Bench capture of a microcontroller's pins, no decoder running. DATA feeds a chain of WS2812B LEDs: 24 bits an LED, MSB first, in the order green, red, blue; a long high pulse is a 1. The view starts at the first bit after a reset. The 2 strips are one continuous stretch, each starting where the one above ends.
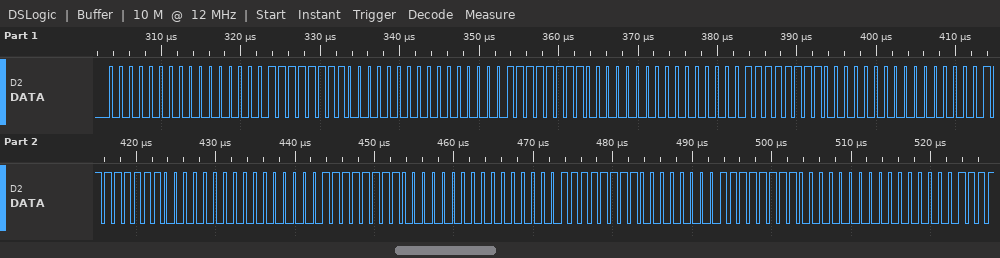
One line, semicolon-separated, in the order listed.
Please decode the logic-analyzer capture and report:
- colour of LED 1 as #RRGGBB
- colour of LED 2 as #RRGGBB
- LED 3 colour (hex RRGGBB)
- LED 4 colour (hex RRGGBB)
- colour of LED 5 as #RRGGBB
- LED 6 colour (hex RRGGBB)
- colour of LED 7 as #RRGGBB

#0000FF; #0000FF; #0000FF; #0000FF; #0000FF; #0000FF; #FF0000
